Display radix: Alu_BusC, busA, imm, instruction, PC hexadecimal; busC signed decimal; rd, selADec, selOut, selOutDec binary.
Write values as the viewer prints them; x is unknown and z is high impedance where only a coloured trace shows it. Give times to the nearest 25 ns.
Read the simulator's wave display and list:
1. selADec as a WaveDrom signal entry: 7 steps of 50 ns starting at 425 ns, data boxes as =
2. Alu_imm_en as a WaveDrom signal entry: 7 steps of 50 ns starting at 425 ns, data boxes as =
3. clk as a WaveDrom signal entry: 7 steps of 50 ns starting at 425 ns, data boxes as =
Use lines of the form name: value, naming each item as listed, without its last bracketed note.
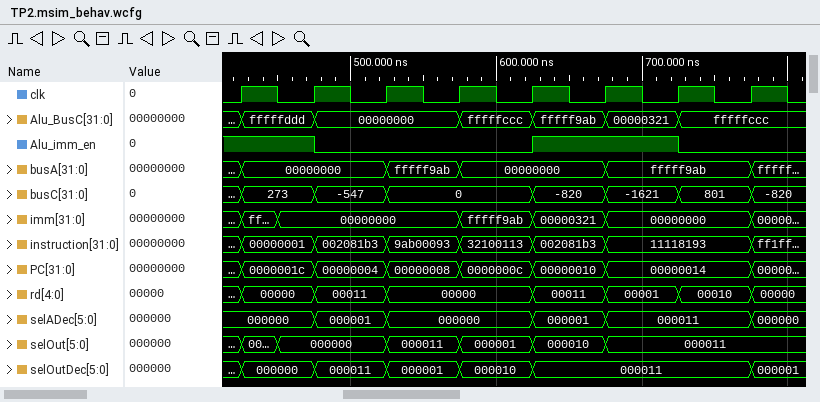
selADec as a WaveDrom signal entry: 7 steps of 50 ns starting at 425 ns, data boxes as =: {name: 'selADec', wave: '===.==.', data: '000000 000001 000000 000001 000011'}
Alu_imm_en as a WaveDrom signal entry: 7 steps of 50 ns starting at 425 ns, data boxes as =: {name: 'Alu_imm_en', wave: '10..1.0'}
clk as a WaveDrom signal entry: 7 steps of 50 ns starting at 425 ns, data boxes as =: {name: 'clk', wave: 'p......'}
